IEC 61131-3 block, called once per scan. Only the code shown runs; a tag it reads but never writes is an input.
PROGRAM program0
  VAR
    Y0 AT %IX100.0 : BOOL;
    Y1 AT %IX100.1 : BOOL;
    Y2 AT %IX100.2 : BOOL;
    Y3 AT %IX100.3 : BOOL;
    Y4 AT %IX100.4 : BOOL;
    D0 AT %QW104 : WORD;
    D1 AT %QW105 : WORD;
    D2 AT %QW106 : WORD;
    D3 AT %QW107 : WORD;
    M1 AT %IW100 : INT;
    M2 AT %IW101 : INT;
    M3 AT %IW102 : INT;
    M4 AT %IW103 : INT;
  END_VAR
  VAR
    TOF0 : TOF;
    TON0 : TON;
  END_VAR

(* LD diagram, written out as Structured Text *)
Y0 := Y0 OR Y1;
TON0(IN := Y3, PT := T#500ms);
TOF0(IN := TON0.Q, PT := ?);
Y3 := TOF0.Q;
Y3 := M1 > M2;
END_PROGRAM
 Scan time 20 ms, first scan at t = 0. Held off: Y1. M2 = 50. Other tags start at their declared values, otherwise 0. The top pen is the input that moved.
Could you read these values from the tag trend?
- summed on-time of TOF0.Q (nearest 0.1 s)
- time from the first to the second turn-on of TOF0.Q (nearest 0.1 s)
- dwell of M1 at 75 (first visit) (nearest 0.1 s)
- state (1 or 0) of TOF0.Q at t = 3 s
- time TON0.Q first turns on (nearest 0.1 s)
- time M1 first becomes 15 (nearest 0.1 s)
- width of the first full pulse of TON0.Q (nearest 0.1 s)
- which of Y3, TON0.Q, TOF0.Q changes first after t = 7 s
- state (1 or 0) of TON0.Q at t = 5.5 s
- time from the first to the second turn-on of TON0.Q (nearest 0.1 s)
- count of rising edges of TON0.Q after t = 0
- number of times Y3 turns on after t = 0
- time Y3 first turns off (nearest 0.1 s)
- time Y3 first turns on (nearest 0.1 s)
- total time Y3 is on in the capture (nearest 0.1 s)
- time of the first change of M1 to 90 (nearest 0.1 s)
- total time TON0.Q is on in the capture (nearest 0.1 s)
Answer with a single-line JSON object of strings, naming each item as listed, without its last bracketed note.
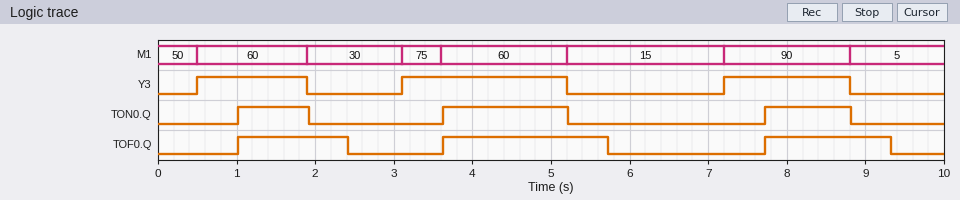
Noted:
{"summed on-time of TOF0.Q": "5.1 s", "time from the first to the second turn-on of TOF0.Q": "2.6 s", "dwell of M1 at 75 (first visit)": "0.5 s", "state (1 or 0) of TOF0.Q at t = 3 s": "0", "time TON0.Q first turns on": "1.0 s", "time M1 first becomes 15": "5.2 s", "width of the first full pulse of TON0.Q": "0.9 s", "which of Y3, TON0.Q, TOF0.Q changes first after t = 7 s": "Y3", "state (1 or 0) of TON0.Q at t = 5.5 s": "0", "time from the first to the second turn-on of TON0.Q": "2.6 s", "count of rising edges of TON0.Q after t = 0": "3", "number of times Y3 turns on after t = 0": "3", "time Y3 first turns off": "1.9 s", "time Y3 first turns on": "0.5 s", "total time Y3 is on in the capture": "5.1 s", "time of the first change of M1 to 90": "7.2 s", "total time TON0.Q is on in the capture": "3.6 s"}
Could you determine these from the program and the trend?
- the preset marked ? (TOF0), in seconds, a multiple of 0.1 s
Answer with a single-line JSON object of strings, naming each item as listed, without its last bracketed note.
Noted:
{"the preset marked ? (TOF0), in seconds, a multiple of 0.1 s": "0.5 s"}
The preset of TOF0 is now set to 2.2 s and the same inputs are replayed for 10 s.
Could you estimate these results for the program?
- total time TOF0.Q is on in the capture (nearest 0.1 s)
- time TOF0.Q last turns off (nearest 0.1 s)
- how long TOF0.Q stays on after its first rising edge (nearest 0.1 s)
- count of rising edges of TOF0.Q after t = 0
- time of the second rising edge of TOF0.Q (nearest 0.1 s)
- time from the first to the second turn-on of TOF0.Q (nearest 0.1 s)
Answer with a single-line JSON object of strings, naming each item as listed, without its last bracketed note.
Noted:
{"total time TOF0.Q is on in the capture": "8.7 s", "time TOF0.Q last turns off": "7.4 s", "how long TOF0.Q stays on after its first rising edge": "6.4 s", "count of rising edges of TOF0.Q after t = 0": "2", "time of the second rising edge of TOF0.Q": "7.7 s", "time from the first to the second turn-on of TOF0.Q": "6.7 s"}
